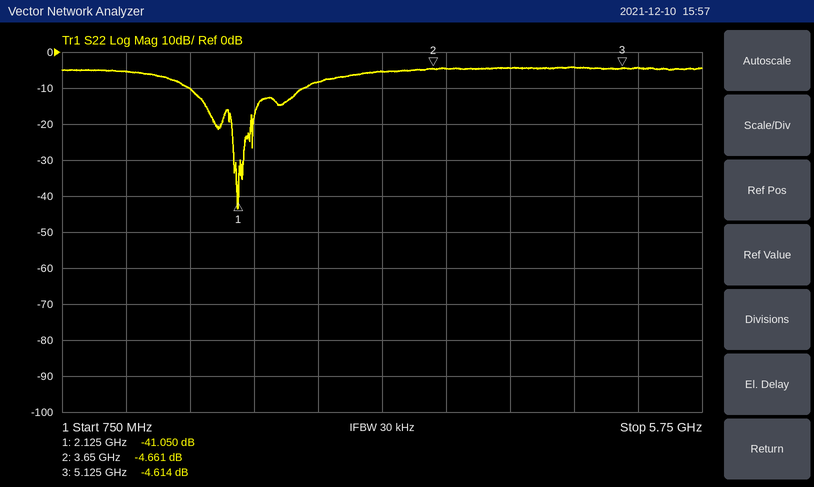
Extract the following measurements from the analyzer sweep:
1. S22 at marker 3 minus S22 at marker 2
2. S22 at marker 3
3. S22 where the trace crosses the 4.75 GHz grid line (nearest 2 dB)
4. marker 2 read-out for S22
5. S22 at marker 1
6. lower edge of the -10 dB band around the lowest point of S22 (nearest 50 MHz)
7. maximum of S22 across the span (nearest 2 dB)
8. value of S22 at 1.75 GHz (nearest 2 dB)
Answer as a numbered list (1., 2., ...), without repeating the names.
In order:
1. 0.047 dB
2. -4.614 dB
3. -4 dB
4. -4.661 dB
5. -41.050 dB
6. 1.75 GHz
7. -4 dB
8. -10 dB
